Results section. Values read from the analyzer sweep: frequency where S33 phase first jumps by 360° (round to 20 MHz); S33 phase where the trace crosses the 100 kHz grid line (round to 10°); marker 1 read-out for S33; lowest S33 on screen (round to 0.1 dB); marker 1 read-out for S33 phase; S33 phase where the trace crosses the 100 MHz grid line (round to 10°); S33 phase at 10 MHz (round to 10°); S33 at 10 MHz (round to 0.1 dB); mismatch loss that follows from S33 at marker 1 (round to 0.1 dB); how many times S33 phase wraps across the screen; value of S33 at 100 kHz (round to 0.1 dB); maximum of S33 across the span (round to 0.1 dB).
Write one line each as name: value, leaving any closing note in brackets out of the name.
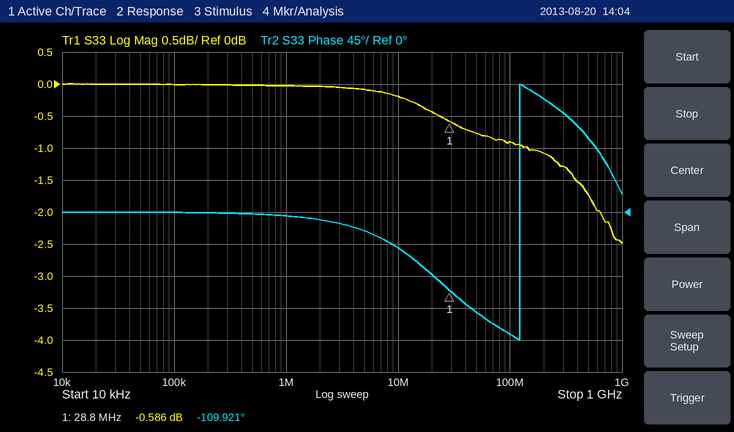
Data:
frequency where S33 phase first jumps by 360°: 120 MHz
S33 phase where the trace crosses the 100 kHz grid line: 0°
marker 1 read-out for S33: -0.586 dB
lowest S33 on screen: -2.5 dB
marker 1 read-out for S33 phase: -109.921°
S33 phase where the trace crosses the 100 MHz grid line: -170°
S33 phase at 10 MHz: -50°
S33 at 10 MHz: -0.2 dB
mismatch loss that follows from S33 at marker 1: 9.0 dB
how many times S33 phase wraps across the screen: 1
value of S33 at 100 kHz: 0.0 dB
maximum of S33 across the span: 0.0 dB
